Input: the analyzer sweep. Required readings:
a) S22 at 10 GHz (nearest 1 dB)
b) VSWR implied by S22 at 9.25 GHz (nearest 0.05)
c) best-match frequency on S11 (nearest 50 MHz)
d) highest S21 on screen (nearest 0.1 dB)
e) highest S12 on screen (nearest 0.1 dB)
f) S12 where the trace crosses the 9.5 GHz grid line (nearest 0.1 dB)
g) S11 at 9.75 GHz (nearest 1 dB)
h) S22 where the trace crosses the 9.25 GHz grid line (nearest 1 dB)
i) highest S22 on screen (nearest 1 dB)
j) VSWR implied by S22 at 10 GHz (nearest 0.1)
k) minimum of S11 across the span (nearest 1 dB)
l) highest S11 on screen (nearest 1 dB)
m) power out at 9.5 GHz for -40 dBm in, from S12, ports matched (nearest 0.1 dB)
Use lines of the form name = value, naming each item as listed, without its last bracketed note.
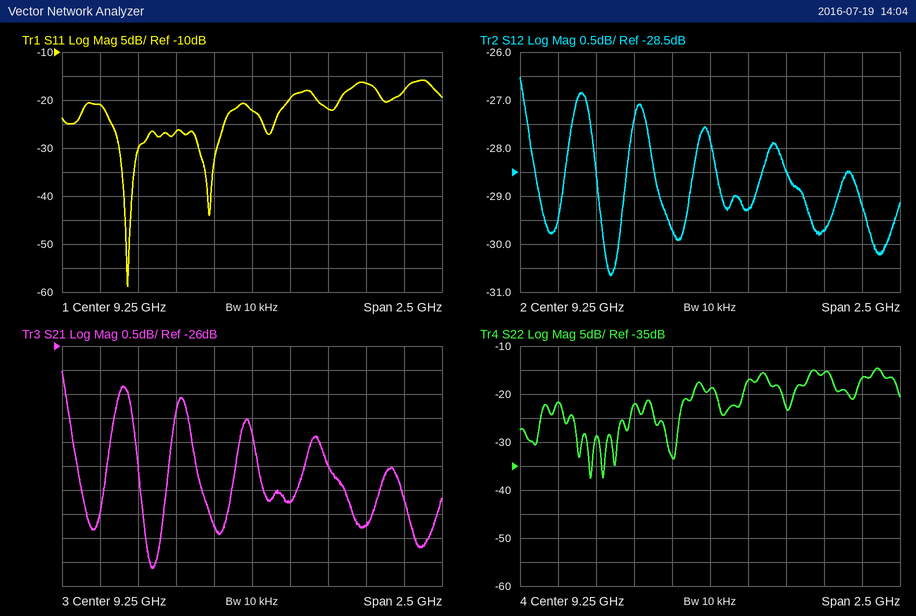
S22 at 10 GHz = -16 dB
VSWR implied by S22 at 9.25 GHz = 1.25
best-match frequency on S11 = 8.45 GHz
highest S21 on screen = -26.5 dB
highest S12 on screen = -26.5 dB
S12 where the trace crosses the 9.5 GHz grid line = -29.3 dB
S11 at 9.75 GHz = -22 dB
S22 where the trace crosses the 9.25 GHz grid line = -19 dB
highest S22 on screen = -15 dB
VSWR implied by S22 at 10 GHz = 1.4
minimum of S11 across the span = -59 dB
highest S11 on screen = -16 dB
power out at 9.5 GHz for -40 dBm in, from S12, ports matched = -69.3 dBm
